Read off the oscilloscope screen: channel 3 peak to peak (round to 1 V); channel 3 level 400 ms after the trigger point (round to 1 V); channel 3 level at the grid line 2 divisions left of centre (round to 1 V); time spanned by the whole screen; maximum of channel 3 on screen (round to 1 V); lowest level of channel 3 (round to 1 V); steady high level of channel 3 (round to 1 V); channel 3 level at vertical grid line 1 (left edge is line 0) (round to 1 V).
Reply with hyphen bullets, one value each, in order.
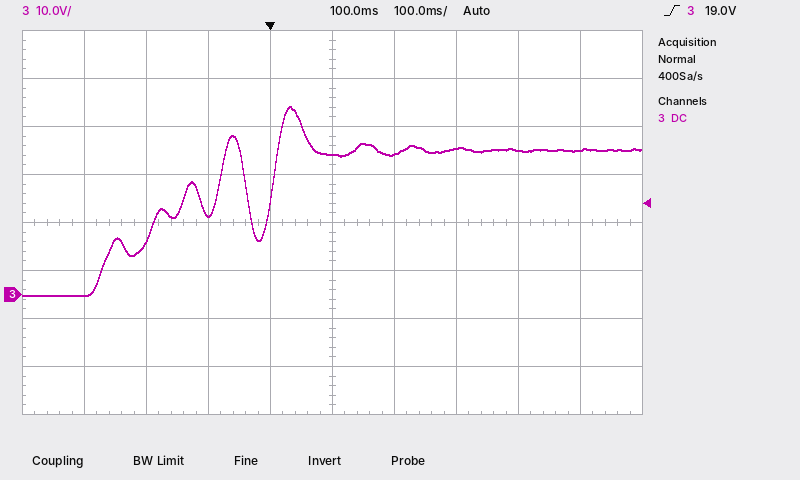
- 39 V
- 30 V
- 17 V
- 1 s
- 39 V
- 0 V
- 30 V
- 0 V
